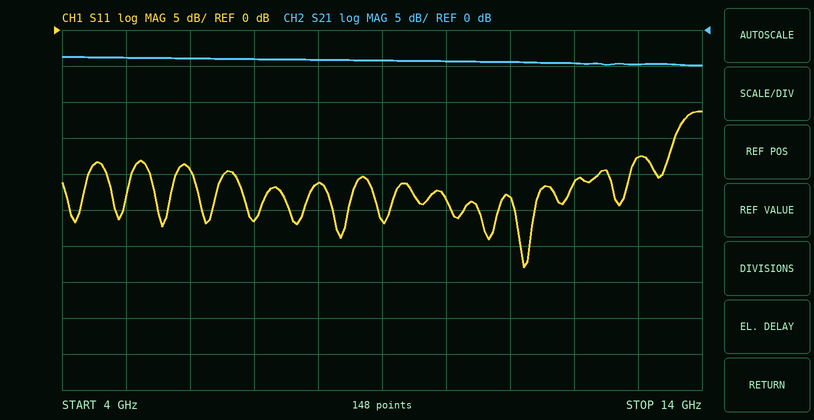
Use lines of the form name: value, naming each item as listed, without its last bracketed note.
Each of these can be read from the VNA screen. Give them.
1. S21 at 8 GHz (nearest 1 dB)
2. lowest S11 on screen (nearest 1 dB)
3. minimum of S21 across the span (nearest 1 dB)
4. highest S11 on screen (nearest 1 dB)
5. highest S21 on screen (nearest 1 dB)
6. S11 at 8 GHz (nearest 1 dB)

S21 at 8 GHz: -4 dB
lowest S11 on screen: -33 dB
minimum of S21 across the span: -5 dB
highest S11 on screen: -11 dB
highest S21 on screen: -4 dB
S11 at 8 GHz: -21 dB
